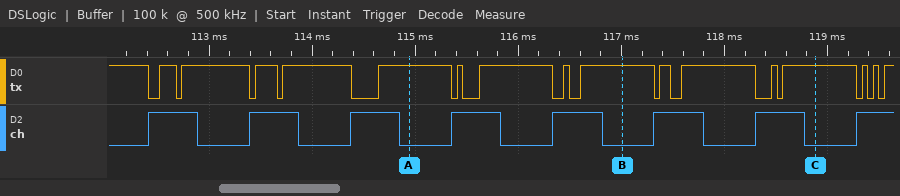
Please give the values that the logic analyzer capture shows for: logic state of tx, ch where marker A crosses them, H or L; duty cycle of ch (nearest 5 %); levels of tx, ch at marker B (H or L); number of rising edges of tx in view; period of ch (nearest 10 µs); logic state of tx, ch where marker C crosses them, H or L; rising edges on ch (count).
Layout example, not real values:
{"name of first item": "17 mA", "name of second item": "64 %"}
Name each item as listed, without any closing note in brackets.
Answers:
{"logic state of tx, ch where marker A crosses them, H or L": "tx=H, ch=L", "duty cycle of ch": "50 %", "levels of tx, ch at marker B": "tx=H, ch=L", "number of rising edges of tx in view": "16", "period of ch": "980 µs", "logic state of tx, ch where marker C crosses them, H or L": "tx=H, ch=L", "rising edges on ch": "8"}
